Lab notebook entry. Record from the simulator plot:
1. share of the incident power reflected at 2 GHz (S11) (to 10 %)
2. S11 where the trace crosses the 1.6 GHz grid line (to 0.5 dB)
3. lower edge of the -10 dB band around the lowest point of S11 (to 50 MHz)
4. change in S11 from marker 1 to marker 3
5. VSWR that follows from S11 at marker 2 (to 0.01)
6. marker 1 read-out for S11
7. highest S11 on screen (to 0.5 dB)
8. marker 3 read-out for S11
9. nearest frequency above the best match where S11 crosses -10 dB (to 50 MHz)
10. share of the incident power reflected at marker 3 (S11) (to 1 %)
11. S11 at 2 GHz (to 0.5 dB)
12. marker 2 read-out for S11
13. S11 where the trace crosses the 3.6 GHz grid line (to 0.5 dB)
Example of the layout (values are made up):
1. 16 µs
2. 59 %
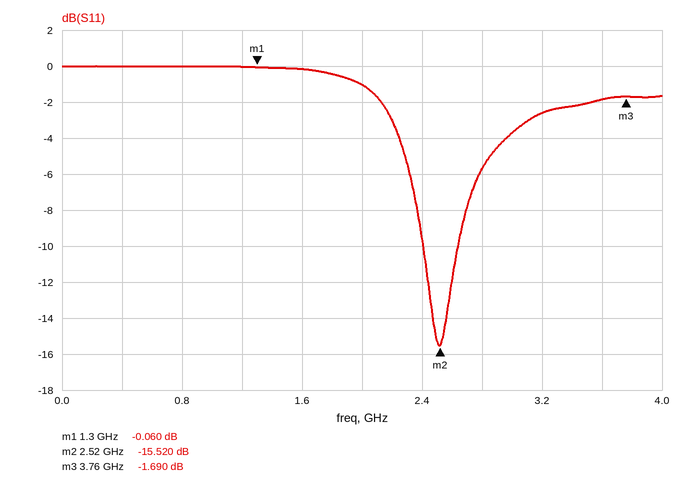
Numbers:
1. 80 %
2. 0.0 dB
3. 2.40 GHz
4. -1.630 dB
5. 1.40
6. -0.060 dB
7. 0.0 dB
8. -1.690 dB
9. 2.65 GHz
10. 68 %
11. -1.0 dB
12. -15.520 dB
13. -2.0 dB
